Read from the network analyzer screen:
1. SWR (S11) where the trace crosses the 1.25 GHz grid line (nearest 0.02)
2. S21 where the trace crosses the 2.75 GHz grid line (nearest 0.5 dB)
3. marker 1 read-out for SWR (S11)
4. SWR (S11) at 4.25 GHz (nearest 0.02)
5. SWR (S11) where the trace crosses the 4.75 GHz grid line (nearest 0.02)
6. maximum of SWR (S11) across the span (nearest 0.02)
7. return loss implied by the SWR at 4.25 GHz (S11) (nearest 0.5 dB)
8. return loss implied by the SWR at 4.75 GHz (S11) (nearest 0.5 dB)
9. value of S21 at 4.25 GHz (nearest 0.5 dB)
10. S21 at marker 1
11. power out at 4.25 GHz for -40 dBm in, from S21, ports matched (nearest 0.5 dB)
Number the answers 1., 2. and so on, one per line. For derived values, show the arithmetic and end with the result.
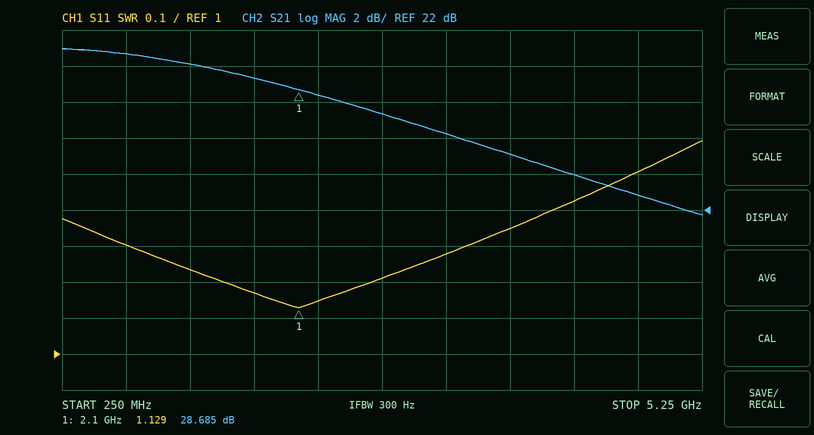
1. 1.24
2. 27.5 dB
3. 1.129
4. 1.42
5. 1.50
6. 1.60
7. −20 log10((1.42 − 1)/(1.42 + 1)) ≈ 15.2 dB, so 15.0 dB to the nearest 0.5 dB
8. −20 log10((1.5 − 1)/(1.5 + 1)) ≈ 14.0 dB
9. 24.0 dB
10. 28.685 dB
11. -40 dBm + (24.0 dB) = -16.0 dBm
